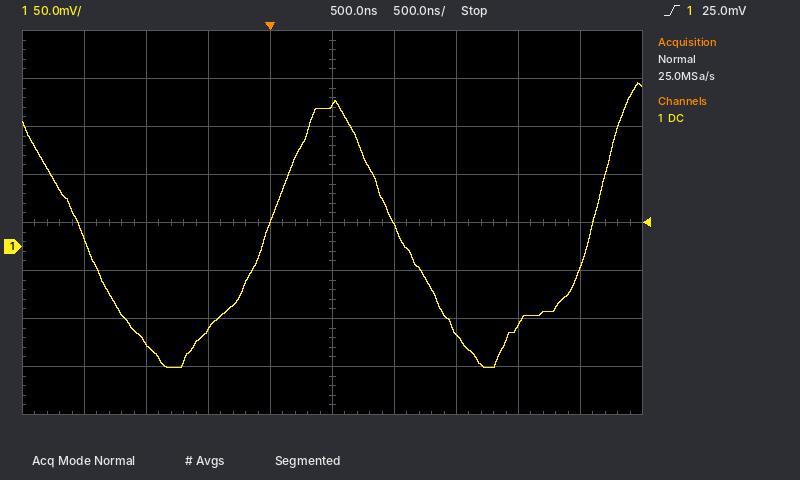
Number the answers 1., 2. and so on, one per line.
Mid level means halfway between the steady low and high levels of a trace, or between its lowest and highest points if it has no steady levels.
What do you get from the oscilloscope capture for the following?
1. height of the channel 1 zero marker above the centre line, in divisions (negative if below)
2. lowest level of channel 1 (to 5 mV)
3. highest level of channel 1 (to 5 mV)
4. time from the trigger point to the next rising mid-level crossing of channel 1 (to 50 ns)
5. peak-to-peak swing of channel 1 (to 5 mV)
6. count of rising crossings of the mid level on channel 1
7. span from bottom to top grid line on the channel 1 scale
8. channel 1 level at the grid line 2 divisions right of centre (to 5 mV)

1. -0.5 div
2. -125 mV
3. 170 mV
4. 2.60 µs
5. 295 mV
6. 2
7. 400 mV
8. -90 mV
